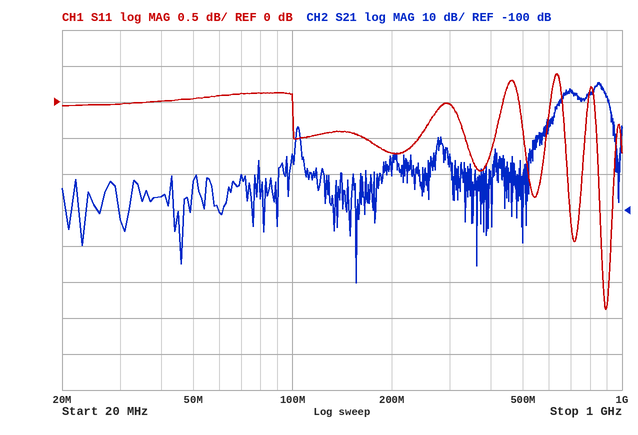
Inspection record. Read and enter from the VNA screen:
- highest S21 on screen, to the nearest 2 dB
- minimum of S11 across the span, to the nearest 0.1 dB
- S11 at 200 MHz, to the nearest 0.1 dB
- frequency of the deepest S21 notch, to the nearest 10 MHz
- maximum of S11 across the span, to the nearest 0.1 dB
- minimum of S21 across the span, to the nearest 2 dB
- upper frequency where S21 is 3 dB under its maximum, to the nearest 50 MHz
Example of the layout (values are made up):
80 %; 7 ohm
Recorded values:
-64 dB; -2.9 dB; -0.7 dB; 160 MHz; 0.4 dB; -120 dB; 900 MHz
